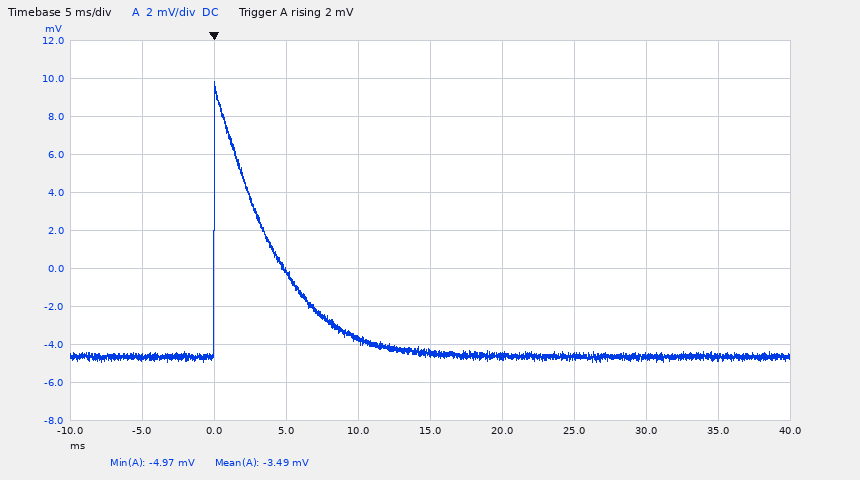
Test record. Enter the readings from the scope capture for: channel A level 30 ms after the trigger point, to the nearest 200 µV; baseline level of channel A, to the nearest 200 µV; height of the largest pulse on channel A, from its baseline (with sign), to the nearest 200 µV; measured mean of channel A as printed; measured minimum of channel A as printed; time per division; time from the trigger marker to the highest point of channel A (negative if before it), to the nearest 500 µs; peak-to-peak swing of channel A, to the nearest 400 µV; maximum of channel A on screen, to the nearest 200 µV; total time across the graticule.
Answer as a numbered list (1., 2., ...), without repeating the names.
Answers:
1. -4.6 mV
2. -4.6 mV
3. +14.4 mV
4. -3.49 mV
5. -4.97 mV
6. 5 ms
7. 0.0 ms
8. 14.8 mV
9. 9.8 mV
10. 50 ms
